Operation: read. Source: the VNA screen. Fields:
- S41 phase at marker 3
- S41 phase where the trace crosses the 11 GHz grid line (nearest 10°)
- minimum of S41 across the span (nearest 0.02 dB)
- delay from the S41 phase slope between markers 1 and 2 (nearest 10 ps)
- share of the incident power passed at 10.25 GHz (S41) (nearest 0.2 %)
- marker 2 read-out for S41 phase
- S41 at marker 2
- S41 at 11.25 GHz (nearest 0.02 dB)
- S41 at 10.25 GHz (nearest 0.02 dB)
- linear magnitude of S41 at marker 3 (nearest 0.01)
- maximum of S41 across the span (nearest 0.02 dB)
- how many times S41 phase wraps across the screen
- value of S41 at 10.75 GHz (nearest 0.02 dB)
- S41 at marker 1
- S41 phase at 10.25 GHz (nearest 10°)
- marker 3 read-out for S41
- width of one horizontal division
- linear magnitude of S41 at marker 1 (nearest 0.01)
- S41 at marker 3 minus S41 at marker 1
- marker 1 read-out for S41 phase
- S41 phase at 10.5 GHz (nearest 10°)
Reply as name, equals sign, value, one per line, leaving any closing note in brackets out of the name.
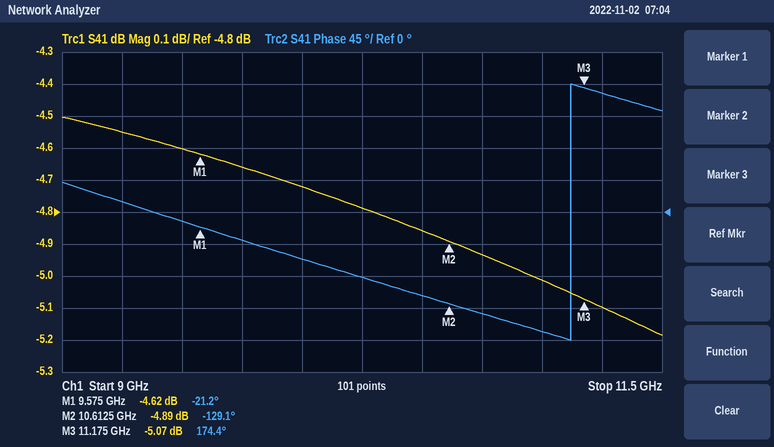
S41 phase at marker 3 = 174.4°
S41 phase where the trace crosses the 11 GHz grid line = -170°
minimum of S41 across the span = -5.18 dB
delay from the S41 phase slope between markers 1 and 2 = 290 ps
share of the incident power passed at 10.25 GHz (S41) = 33.2 %
marker 2 read-out for S41 phase = -129.1°
S41 at marker 2 = -4.89 dB
S41 at 11.25 GHz = -5.10 dB
S41 at 10.25 GHz = -4.78 dB
linear magnitude of S41 at marker 3 = 0.56
maximum of S41 across the span = -4.50 dB
how many times S41 phase wraps across the screen = 1
value of S41 at 10.75 GHz = -4.94 dB
S41 at marker 1 = -4.62 dB
S41 phase at 10.25 GHz = -90°
marker 3 read-out for S41 = -5.07 dB
width of one horizontal division = 250 MHz
linear magnitude of S41 at marker 1 = 0.59
S41 at marker 3 minus S41 at marker 1 = -0.45 dB
marker 1 read-out for S41 phase = -21.2°
S41 phase at 10.5 GHz = -120°
